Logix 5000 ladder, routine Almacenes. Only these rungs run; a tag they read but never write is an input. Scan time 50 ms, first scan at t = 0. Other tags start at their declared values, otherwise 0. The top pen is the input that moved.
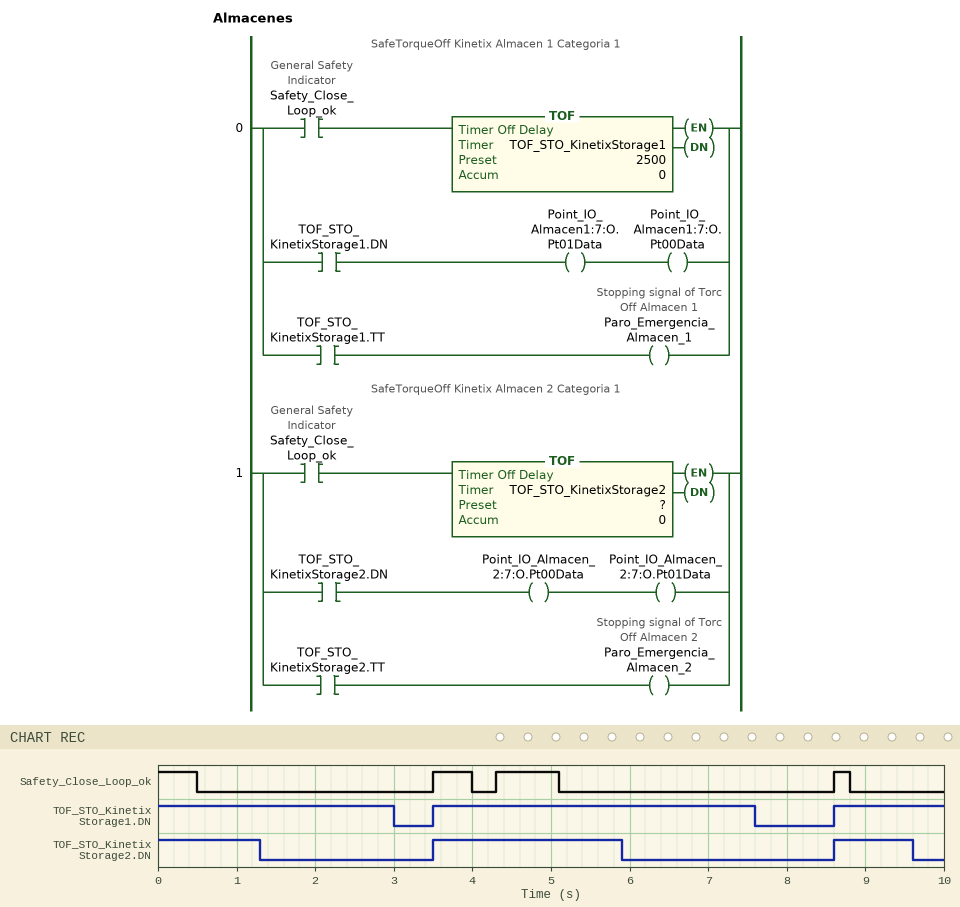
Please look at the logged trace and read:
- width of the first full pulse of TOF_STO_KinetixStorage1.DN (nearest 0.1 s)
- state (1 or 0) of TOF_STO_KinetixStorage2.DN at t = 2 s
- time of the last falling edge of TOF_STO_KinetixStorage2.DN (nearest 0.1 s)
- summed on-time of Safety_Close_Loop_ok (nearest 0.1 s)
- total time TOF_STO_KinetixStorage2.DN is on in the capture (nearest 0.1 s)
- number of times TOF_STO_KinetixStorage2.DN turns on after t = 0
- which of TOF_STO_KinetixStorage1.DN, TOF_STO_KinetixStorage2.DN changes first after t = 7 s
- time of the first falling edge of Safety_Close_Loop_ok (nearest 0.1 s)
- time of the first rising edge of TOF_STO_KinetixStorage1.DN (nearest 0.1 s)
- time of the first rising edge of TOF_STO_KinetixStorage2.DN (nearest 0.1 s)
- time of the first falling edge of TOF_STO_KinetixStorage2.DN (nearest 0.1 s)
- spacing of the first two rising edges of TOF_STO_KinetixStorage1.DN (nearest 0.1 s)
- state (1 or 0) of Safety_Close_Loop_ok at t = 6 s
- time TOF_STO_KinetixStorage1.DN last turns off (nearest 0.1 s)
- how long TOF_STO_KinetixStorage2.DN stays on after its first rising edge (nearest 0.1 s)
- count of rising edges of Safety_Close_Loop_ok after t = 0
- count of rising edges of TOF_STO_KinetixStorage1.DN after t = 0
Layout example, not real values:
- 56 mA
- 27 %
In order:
- 4.1 s
- 0
- 9.6 s
- 2.0 s
- 4.7 s
- 2
- TOF_STO_KinetixStorage1.DN
- 0.5 s
- 3.5 s
- 3.5 s
- 1.3 s
- 5.1 s
- 0
- 7.6 s
- 2.4 s
- 3
- 2
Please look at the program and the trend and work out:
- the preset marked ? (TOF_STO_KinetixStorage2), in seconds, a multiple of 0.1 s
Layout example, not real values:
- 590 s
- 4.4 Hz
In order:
- 0.8 s
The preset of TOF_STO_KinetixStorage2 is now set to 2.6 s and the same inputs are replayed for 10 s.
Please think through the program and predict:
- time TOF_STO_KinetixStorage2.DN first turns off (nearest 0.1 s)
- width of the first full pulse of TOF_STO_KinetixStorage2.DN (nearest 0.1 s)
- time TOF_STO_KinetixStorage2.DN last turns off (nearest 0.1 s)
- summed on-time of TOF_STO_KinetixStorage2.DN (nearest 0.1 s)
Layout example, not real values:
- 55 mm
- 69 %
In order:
- 3.1 s
- 4.2 s
- 7.7 s
- 8.7 s
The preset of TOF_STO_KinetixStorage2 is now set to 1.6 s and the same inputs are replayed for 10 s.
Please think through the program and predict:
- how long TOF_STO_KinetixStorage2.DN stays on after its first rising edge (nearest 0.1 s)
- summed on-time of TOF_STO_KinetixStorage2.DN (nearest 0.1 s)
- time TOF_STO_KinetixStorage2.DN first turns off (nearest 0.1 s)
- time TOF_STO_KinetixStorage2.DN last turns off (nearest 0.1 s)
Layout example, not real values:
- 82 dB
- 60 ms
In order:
- 3.2 s
- 6.7 s
- 2.1 s
- 6.7 s
